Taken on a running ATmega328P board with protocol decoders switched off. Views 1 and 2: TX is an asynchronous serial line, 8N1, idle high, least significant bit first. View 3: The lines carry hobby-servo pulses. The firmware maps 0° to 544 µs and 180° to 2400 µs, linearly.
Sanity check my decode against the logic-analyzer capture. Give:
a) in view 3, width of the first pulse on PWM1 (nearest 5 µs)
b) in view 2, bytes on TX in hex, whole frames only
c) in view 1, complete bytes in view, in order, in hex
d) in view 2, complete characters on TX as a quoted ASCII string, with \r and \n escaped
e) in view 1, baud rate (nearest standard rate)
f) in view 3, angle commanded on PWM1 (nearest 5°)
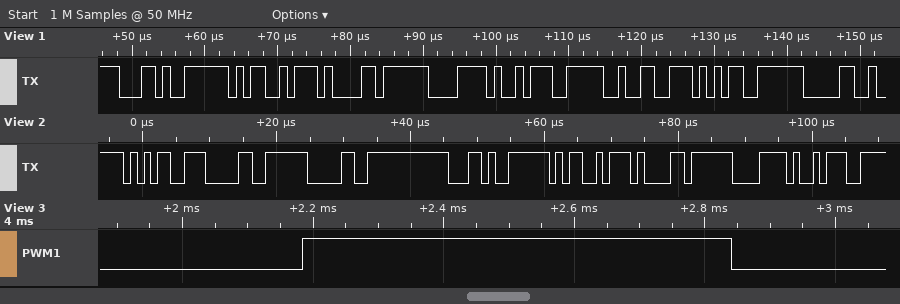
655 µs
35 30 30 2C 4D 61 78 3A
2C 4D 61 78 3A 32 35 30
"500,Max:"
1000000 baud
10°
